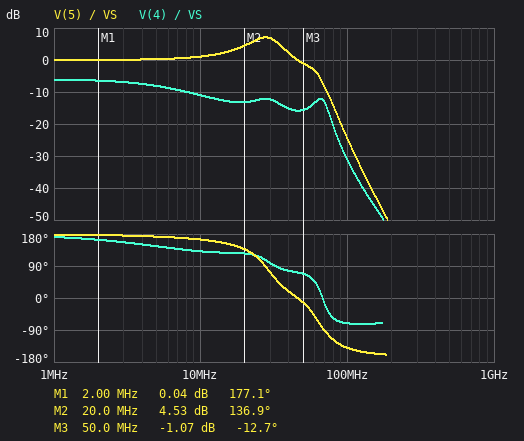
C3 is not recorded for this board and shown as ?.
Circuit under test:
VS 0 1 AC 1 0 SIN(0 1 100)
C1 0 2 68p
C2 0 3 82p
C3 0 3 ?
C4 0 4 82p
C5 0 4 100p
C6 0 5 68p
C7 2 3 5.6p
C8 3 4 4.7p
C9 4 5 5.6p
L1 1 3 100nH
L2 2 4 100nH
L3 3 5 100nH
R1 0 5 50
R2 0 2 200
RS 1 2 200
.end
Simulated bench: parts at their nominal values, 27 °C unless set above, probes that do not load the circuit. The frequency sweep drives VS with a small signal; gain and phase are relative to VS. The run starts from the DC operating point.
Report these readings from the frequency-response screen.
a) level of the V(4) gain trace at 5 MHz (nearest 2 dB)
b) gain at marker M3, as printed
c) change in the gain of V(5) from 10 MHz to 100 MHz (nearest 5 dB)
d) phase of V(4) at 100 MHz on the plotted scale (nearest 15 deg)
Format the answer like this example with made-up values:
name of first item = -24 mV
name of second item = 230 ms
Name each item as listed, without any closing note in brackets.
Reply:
level of the V(4) gain trace at 5 MHz = -8 dB
gain at marker M3, as printed = -1.07 dB
change in the gain of V(5) from 10 MHz to 100 MHz = -25 dB
phase of V(4) at 100 MHz on the plotted scale = -75 deg
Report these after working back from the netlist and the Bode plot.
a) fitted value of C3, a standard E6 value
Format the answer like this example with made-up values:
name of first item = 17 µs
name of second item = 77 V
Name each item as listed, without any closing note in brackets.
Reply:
fitted value of C3, a standard E6 value = 150 pF
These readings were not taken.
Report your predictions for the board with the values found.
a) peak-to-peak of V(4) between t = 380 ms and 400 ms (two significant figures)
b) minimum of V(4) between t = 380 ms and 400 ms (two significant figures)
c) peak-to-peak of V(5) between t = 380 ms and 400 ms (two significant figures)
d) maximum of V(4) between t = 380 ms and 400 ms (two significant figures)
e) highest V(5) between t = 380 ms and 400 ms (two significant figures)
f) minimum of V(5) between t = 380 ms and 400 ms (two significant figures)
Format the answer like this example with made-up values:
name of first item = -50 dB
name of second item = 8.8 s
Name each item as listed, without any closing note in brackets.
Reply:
peak-to-peak of V(4) between t = 380 ms and 400 ms = 1.0 V
minimum of V(4) between t = 380 ms and 400 ms = -500 mV
peak-to-peak of V(5) between t = 380 ms and 400 ms = 2.0 V
maximum of V(4) between t = 380 ms and 400 ms = 500 mV
highest V(5) between t = 380 ms and 400 ms = 1.0 V
minimum of V(5) between t = 380 ms and 400 ms = -1.0 V
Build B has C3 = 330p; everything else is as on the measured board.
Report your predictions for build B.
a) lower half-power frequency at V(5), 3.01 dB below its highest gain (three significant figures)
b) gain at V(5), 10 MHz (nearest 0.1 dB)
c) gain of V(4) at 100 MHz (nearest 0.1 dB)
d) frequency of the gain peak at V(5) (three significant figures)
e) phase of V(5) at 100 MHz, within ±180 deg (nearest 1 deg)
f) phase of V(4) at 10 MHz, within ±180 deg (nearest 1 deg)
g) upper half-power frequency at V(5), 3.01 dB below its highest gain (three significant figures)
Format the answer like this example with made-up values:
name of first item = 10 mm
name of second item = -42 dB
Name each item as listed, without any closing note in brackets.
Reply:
lower half-power frequency at V(5), 3.01 dB below its highest gain = 18.0 MHz
gain at V(5), 10 MHz = 1.8 dB
gain of V(4) at 100 MHz = -31.5 dB
frequency of the gain peak at V(5) = 22.7 MHz
phase of V(5) at 100 MHz, within ±180 deg = -139 deg
phase of V(4) at 10 MHz, within ±180 deg = 132 deg
upper half-power frequency at V(5), 3.01 dB below its highest gain = 27.0 MHz
